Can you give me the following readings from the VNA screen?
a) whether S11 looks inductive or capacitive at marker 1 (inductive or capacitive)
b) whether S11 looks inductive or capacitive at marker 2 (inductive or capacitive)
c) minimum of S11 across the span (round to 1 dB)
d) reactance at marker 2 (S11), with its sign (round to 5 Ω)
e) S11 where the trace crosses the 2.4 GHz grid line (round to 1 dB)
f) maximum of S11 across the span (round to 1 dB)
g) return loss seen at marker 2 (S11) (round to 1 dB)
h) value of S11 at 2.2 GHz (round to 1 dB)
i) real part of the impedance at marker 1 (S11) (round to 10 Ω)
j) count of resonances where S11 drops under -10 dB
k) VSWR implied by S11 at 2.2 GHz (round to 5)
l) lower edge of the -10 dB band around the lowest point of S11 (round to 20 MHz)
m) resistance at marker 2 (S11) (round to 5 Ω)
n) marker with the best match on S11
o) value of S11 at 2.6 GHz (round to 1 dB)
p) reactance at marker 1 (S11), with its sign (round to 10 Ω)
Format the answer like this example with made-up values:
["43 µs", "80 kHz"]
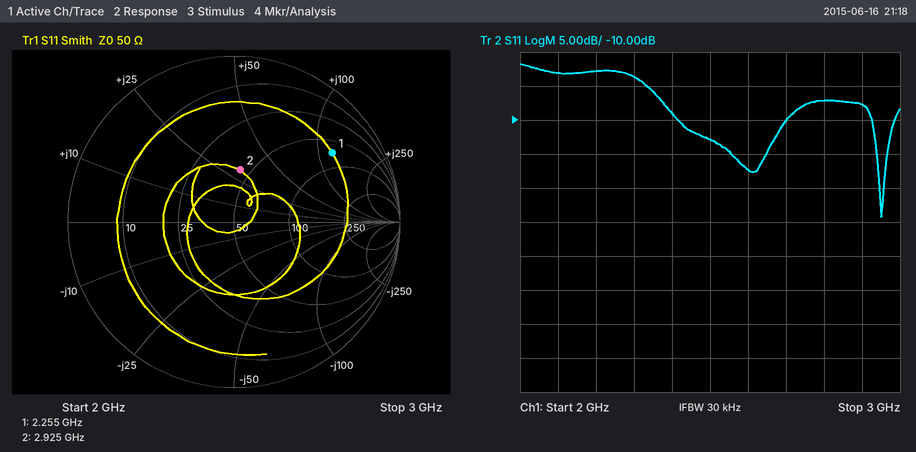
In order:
["inductive", "inductive", "-24 dB", "+30 Ω", "-9 dB", "-2 dB", "10 dB", "-3 dB", "70 Ω", "2", "5", "2.92 GHz", "45 Ω", "marker 2", "-17 dB", "+120 Ω"]
